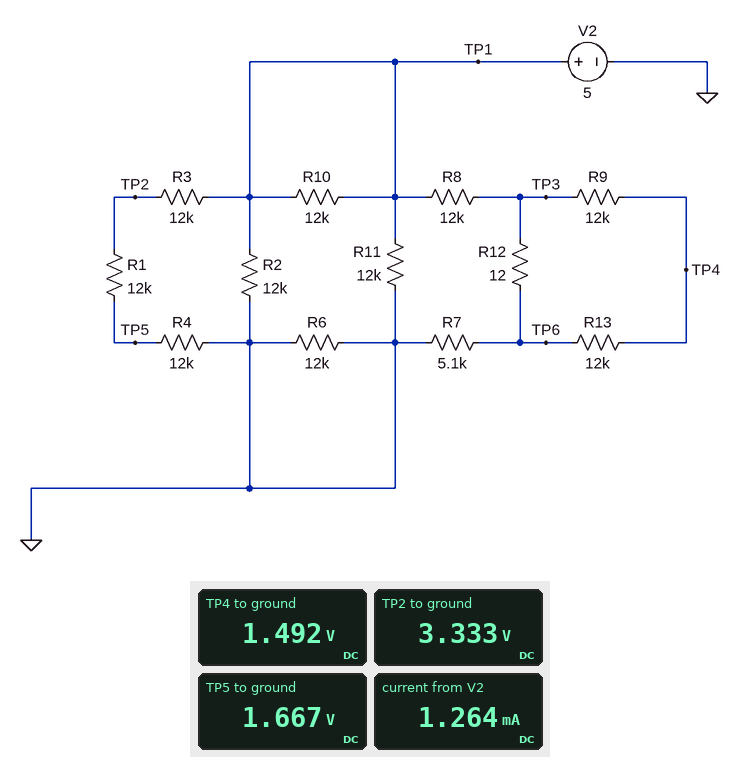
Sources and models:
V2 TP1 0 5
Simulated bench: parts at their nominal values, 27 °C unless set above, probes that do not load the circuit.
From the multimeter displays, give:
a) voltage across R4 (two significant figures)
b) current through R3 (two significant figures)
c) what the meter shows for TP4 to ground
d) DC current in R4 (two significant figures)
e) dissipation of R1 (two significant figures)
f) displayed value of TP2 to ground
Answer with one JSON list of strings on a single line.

["1.7 V", "140 µA", "1.492 V", "140 µA", "230 µW", "3.333 V"]
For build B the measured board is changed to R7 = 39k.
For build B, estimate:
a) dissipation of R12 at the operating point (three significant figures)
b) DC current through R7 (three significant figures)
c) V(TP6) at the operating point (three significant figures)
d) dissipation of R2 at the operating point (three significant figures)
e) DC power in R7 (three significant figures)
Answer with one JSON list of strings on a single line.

["115 nW", "98.0 µA", "3.82 V", "2.08 mW", "375 µW"]
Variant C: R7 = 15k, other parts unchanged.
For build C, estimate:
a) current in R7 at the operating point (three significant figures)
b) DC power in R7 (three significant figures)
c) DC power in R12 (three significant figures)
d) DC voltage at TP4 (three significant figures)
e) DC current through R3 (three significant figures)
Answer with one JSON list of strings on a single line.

["185 µA", "514 µW", "411 nW", "2.78 V", "139 µA"]
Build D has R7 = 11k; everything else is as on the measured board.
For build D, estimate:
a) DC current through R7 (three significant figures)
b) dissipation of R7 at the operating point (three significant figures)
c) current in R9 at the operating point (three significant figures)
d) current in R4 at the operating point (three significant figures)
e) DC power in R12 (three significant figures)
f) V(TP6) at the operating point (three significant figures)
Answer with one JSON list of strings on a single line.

["217 µA", "519 µW", "109 nA", "139 µA", "566 nW", "2.39 V"]
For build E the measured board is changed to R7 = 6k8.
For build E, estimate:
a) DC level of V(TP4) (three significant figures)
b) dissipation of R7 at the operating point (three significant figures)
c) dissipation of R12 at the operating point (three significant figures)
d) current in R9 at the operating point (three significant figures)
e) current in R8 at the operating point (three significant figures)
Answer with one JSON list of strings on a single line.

["1.81 V", "480 µW", "847 nW", "133 nA", "266 µA"]
